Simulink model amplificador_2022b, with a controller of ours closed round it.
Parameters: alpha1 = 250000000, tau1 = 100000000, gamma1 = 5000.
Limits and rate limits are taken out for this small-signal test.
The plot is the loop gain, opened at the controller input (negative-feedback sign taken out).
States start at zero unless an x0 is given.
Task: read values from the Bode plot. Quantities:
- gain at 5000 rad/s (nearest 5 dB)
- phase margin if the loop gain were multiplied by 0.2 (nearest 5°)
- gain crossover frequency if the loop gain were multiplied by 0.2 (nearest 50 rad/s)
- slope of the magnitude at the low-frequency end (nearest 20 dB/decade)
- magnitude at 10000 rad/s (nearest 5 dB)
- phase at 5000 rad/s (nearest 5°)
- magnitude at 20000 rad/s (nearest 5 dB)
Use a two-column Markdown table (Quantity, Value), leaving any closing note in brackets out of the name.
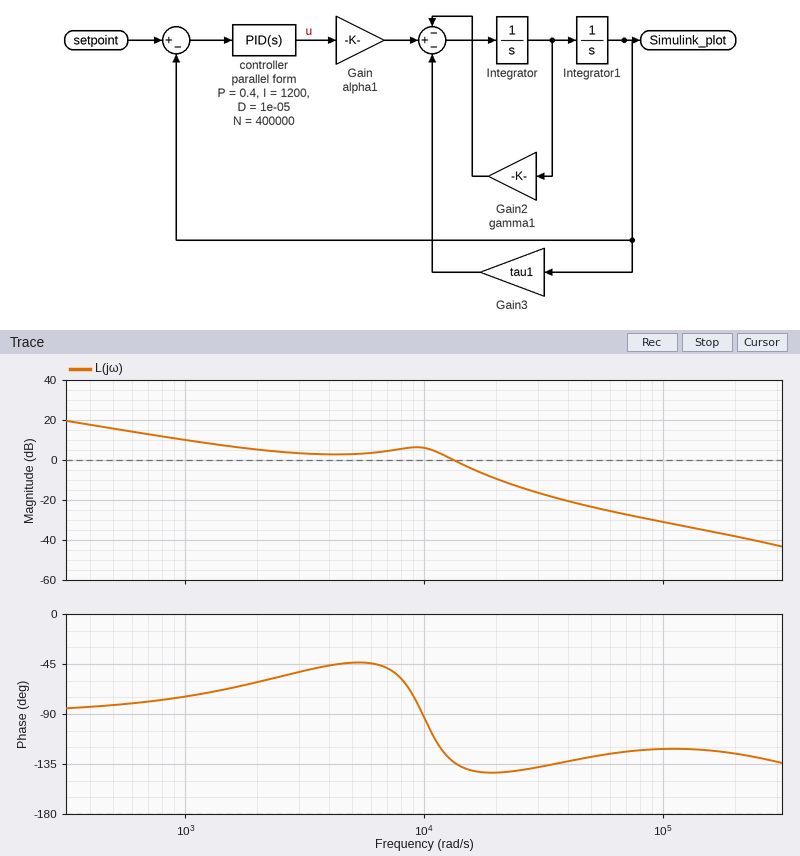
| Quantity | Value |
|---|---|
| gain at 5000 rad/s | 5 dB |
| phase margin if the loop gain were multiplied by 0.2 | 100° |
| gain crossover frequency if the loop gain were multiplied by 0.2 | 600 rad/s |
| slope of the magnitude at the low-frequency end | -20 dB/decade |
| magnitude at 10000 rad/s | 5 dB |
| phase at 5000 rad/s | -45° |
| magnitude at 20000 rad/s | -10 dB |
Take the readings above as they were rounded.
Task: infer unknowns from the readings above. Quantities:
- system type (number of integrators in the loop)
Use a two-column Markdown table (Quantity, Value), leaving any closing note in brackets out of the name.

| Quantity | Value |
|---|---|
| system type | 1 |
